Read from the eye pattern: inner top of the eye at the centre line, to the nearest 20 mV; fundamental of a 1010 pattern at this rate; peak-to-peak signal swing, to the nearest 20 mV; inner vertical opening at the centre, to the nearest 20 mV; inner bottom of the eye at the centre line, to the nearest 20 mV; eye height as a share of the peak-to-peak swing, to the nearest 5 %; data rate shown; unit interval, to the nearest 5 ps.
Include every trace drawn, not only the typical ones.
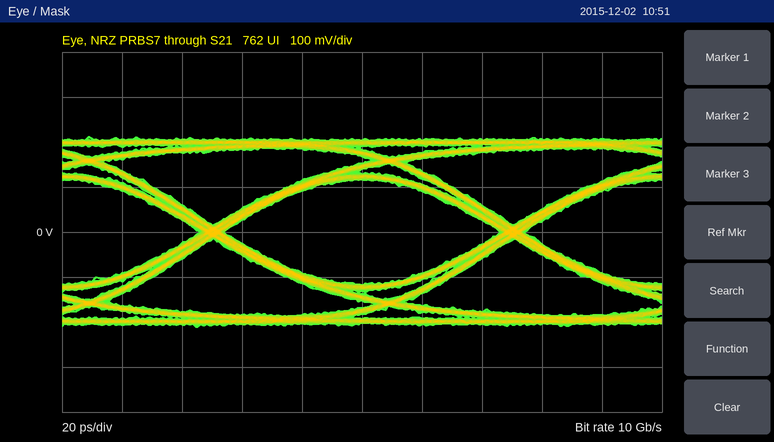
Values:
120 mV
5 GHz
420 mV
240 mV
-120 mV
55 %
10 Gb/s
100 ps
